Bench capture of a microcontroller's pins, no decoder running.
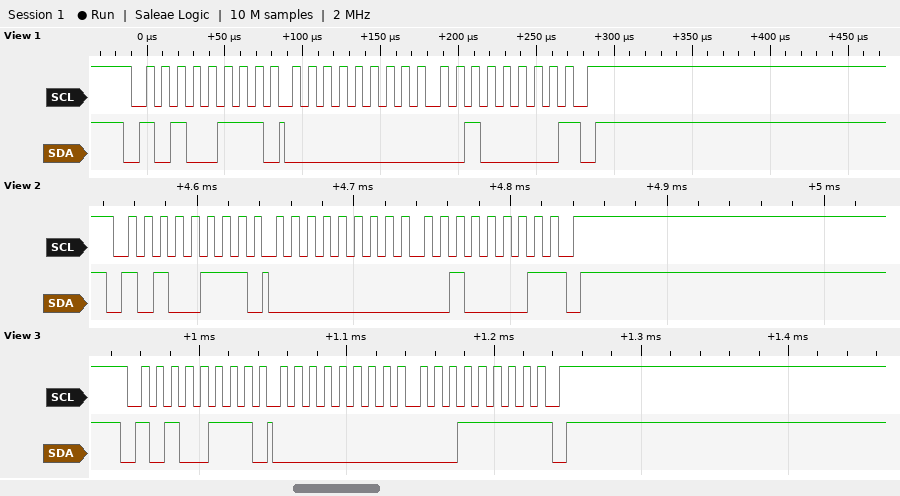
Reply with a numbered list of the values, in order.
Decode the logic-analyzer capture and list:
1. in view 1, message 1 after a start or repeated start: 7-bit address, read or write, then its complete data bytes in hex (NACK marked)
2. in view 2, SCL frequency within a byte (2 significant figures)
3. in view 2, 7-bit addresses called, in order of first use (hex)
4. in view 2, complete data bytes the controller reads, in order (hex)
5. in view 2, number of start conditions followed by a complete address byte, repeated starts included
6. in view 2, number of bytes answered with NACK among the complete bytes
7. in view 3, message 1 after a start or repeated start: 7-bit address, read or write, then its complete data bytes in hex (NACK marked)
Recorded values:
1. 0x53 read: 00 20 NACK
2. 100 kHz
3. 0x53
4. 00 21
5. 1
6. 1
7. 0x53 read: 00 1F NACK
